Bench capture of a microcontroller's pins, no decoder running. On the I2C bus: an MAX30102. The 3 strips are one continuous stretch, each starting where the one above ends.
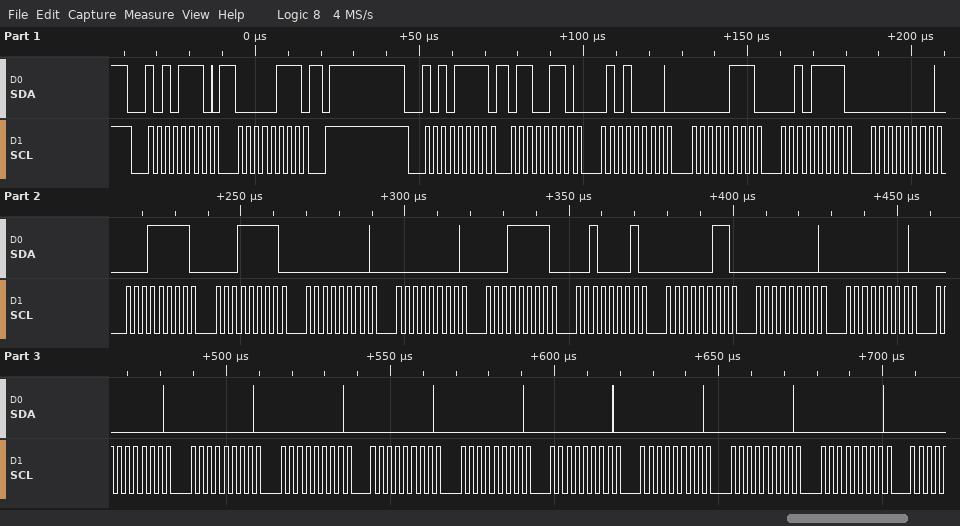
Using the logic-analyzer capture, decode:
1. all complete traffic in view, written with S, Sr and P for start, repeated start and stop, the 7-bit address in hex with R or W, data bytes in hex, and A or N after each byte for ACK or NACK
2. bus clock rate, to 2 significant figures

S 57W A 07 A P S 57R A 66 A 50 A 07 A 2F A 00 A 1F A 1F A 00 A 00 A 1F A 21 A 03 A 00 A 00 A 00 A 00 A 00 A 00 A 00 A 00 A 00 A 00 A 00 A
400 kHz
